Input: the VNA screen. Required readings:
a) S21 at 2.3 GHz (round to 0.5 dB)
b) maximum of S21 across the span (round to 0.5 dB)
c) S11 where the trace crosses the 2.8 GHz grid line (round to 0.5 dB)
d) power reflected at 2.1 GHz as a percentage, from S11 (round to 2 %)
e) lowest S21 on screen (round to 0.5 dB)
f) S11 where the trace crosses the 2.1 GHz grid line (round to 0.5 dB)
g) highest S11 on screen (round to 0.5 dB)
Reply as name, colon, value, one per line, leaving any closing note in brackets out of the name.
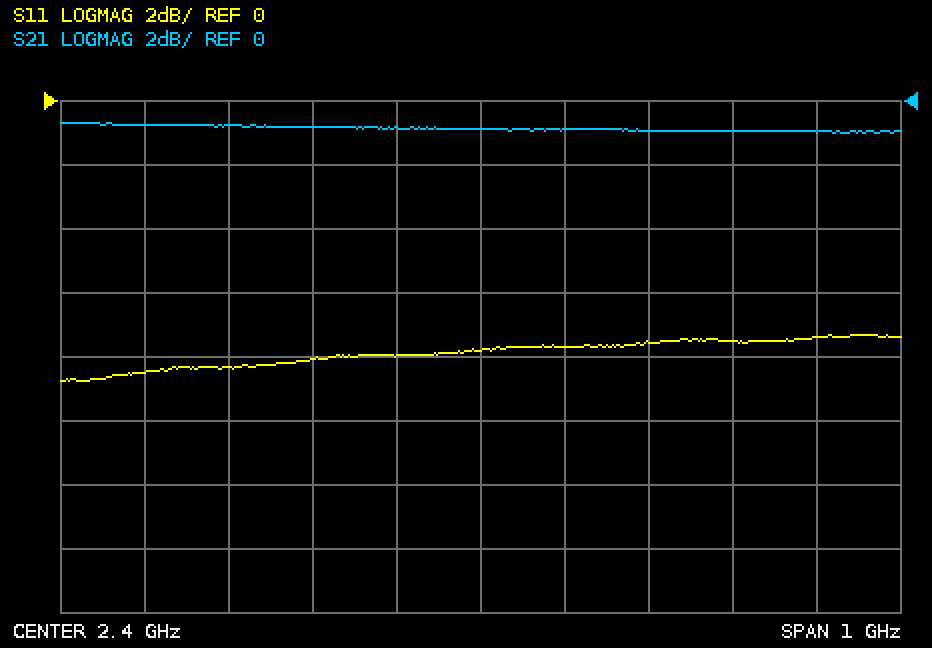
S21 at 2.3 GHz: -1.0 dB
maximum of S21 across the span: -0.5 dB
S11 where the trace crosses the 2.8 GHz grid line: -7.5 dB
power reflected at 2.1 GHz as a percentage, from S11: 14 %
lowest S21 on screen: -1.0 dB
S11 where the trace crosses the 2.1 GHz grid line: -8.5 dB
highest S11 on screen: -7.5 dB
